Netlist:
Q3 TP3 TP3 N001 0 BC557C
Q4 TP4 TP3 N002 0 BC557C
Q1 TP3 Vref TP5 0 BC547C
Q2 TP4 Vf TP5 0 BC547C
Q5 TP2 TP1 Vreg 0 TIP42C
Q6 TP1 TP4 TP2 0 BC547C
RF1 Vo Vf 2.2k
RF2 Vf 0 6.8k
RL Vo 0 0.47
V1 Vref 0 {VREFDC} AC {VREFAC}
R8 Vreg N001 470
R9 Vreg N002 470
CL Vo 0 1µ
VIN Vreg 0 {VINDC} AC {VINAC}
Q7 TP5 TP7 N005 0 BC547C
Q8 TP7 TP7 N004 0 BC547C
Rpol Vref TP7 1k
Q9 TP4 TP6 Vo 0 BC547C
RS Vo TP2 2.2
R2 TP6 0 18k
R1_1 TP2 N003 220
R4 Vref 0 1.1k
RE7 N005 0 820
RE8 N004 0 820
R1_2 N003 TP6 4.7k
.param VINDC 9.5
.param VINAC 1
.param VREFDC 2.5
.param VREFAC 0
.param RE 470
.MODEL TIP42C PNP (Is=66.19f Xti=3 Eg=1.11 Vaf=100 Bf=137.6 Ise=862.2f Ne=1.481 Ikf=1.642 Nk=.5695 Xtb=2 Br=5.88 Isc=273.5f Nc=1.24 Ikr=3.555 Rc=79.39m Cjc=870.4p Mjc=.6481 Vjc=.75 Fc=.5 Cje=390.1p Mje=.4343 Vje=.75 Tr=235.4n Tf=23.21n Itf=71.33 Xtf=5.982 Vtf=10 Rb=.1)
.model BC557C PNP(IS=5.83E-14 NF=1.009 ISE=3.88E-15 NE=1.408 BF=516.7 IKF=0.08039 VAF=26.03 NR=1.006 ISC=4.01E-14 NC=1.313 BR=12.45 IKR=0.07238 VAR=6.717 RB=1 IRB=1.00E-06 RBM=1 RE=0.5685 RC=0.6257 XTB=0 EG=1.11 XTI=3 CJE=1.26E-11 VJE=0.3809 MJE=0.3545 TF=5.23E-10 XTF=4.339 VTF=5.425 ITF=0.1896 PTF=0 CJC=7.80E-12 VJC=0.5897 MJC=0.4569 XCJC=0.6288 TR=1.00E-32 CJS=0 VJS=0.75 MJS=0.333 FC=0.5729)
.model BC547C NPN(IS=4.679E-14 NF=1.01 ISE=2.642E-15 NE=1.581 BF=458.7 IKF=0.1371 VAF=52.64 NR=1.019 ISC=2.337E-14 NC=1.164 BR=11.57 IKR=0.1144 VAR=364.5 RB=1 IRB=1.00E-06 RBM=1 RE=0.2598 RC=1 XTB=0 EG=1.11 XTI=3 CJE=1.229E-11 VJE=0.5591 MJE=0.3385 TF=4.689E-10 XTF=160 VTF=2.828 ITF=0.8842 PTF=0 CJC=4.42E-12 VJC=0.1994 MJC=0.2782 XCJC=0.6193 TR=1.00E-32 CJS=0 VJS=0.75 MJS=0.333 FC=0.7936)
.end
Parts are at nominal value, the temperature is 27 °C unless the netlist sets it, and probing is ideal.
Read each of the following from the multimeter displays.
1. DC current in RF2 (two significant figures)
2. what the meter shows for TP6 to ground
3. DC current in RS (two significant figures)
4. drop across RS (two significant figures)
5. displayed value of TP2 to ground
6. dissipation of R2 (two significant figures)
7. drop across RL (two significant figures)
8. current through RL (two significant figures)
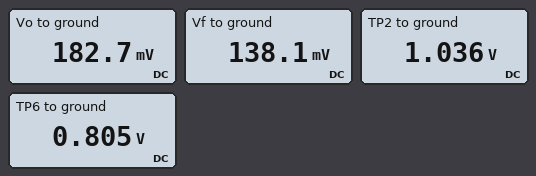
20 µA
0.805 V
390 mA
850 mV
1.036 V
36 µW
180 mV
390 mA
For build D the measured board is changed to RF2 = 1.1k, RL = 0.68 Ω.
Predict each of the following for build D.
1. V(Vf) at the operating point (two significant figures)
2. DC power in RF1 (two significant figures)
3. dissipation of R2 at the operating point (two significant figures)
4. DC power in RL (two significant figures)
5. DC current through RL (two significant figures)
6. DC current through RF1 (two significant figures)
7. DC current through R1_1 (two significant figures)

91 mV
15 µW
44 µW
110 mW
400 mA
82 µA
52 µA
